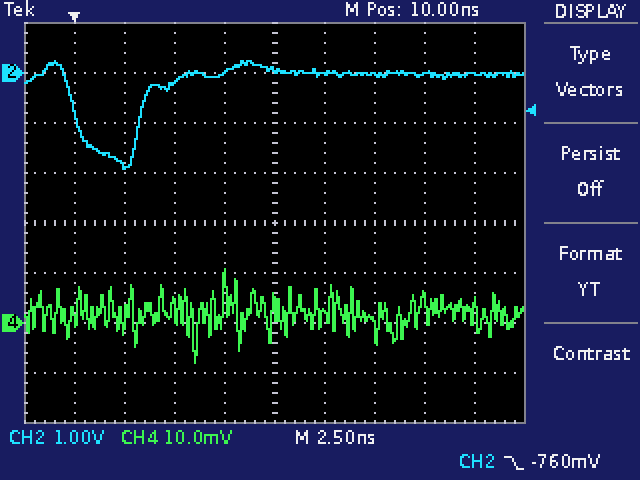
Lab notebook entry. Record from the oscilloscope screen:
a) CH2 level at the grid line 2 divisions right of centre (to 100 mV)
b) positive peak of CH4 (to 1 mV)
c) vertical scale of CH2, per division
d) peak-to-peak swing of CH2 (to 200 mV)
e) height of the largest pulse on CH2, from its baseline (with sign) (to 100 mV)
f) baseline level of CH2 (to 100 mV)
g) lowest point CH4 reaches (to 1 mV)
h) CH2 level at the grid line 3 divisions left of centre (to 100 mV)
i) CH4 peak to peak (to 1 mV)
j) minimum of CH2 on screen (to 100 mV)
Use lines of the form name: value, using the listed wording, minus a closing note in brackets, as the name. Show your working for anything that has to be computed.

CH2 level at the grid line 2 divisions right of centre: 0.0 V
positive peak of CH4: 11 mV
vertical scale of CH2, per division: 1 V
peak-to-peak swing of CH2: 2.2 V
height of the largest pulse on CH2, from its baseline (with sign): -1.9 V − (0.0 V) = -1.9 V
baseline level of CH2: 0.0 V
lowest point CH4 reaches: -8 mV
CH2 level at the grid line 3 divisions left of centre: -1.8 V
CH4 peak to peak: 11 mV − (-8 mV) = 19 mV
minimum of CH2 on screen: -1.9 V
